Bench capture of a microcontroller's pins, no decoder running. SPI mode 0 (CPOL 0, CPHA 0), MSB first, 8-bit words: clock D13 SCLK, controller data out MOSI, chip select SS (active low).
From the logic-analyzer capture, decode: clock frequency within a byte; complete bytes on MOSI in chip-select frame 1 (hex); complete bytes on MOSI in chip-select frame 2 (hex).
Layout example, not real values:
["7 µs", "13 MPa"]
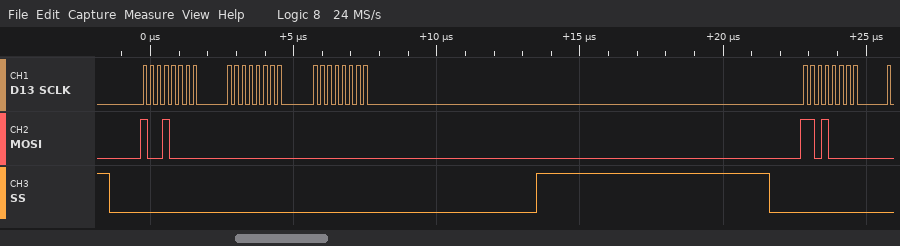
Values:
["4 MHz", "90 00 00", "D0"]
